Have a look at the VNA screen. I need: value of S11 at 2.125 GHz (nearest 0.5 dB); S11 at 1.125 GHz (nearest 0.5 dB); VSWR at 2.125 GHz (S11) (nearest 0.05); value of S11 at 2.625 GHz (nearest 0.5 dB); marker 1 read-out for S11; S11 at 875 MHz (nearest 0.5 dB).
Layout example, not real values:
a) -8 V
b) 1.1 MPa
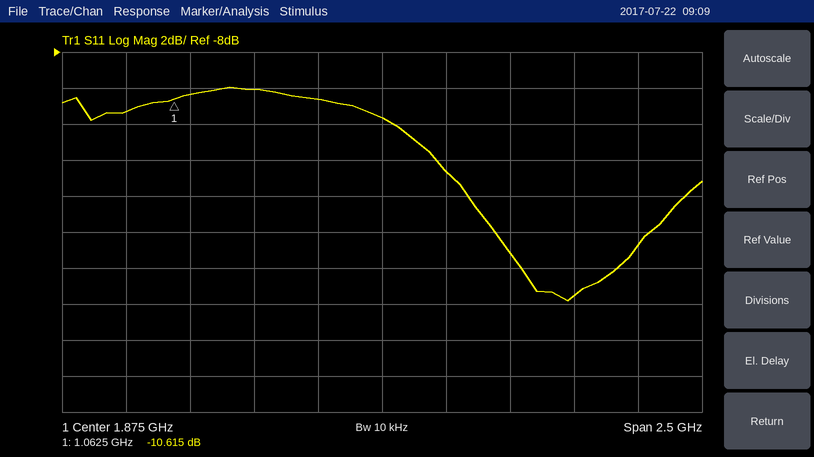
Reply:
a) -14.5 dB
b) -10.5 dB
c) 1.45
d) -21.5 dB
e) -10.615 dB
f) -11.5 dB
